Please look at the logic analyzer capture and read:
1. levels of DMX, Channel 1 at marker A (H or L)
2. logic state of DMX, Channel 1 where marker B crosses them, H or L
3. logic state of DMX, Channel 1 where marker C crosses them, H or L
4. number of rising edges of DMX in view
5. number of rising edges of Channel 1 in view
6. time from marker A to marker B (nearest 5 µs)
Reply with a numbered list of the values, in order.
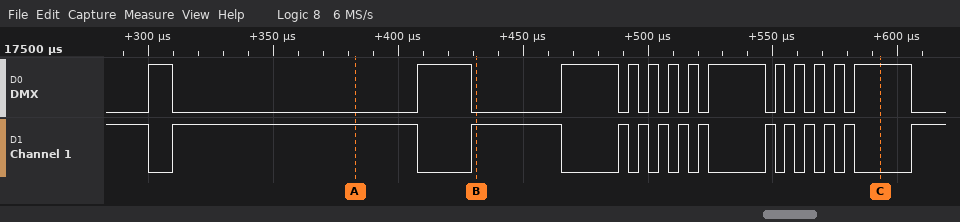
1. DMX=L, Channel 1=H
2. DMX=L, Channel 1=H
3. DMX=H, Channel 1=L
4. 13
5. 13
6. 50 µs
